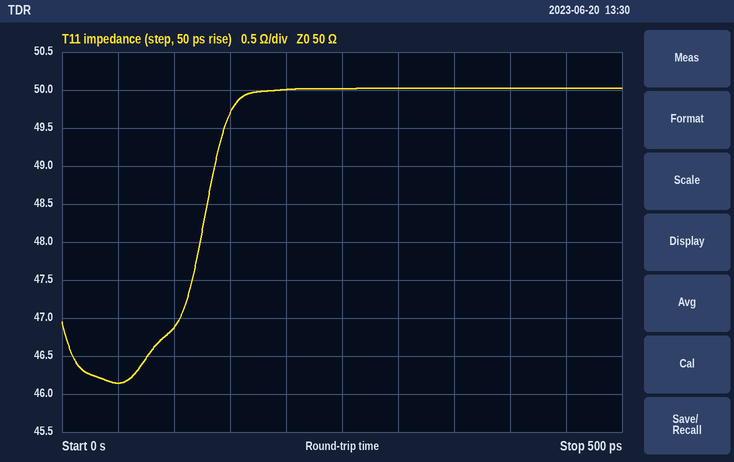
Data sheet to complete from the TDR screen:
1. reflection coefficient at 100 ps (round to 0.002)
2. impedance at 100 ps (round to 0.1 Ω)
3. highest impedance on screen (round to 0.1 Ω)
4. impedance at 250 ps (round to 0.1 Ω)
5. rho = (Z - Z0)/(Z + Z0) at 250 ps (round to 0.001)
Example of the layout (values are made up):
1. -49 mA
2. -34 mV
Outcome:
1. -0.032
2. 46.9 Ω
3. 50.0 Ω
4. 50.0 Ω
5. 0.000
